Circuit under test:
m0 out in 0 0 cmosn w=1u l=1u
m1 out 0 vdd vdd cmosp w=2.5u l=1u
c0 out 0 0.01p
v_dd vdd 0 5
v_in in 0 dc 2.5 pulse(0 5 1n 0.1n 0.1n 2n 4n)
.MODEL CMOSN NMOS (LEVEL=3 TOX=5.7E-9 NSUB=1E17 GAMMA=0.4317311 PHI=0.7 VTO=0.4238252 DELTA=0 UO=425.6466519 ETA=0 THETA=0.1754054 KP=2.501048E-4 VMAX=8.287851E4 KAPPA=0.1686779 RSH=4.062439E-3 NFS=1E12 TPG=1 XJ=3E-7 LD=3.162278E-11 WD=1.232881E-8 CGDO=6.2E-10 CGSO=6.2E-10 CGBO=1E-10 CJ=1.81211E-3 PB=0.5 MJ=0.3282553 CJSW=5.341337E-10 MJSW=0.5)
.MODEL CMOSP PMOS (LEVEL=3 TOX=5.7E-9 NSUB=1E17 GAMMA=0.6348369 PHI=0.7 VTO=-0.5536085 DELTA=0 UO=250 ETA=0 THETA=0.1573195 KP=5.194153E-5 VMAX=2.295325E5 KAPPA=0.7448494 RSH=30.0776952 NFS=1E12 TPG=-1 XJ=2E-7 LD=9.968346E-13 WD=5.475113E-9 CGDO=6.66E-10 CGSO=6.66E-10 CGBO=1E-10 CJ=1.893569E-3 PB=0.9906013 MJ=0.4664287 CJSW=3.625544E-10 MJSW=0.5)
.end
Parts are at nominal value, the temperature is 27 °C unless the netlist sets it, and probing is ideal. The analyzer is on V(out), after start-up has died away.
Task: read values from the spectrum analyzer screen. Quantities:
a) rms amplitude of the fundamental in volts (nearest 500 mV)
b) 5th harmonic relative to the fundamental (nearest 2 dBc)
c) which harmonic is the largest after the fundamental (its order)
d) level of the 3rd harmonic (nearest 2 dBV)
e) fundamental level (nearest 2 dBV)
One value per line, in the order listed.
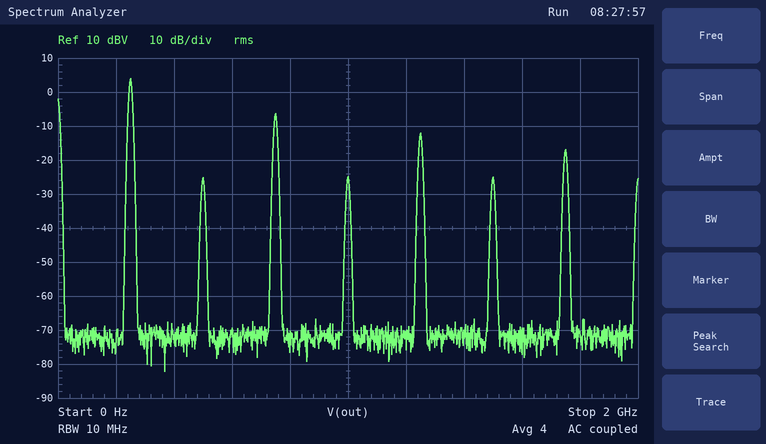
1.5 V
-16 dBc
3
-6 dBV
4 dBV
